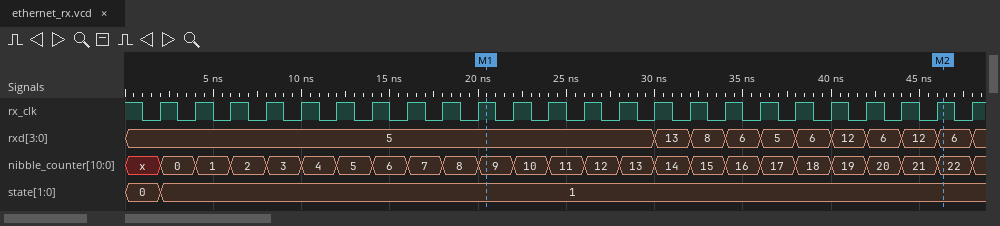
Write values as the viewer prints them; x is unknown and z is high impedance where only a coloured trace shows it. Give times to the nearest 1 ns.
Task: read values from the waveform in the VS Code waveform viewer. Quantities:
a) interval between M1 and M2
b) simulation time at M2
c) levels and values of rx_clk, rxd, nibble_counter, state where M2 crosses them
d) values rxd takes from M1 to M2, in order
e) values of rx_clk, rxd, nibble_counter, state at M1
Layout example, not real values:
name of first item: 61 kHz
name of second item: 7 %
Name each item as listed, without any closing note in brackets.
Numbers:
interval between M1 and M2: 26 ns
simulation time at M2: 46 ns
levels and values of rx_clk, rxd, nibble_counter, state where M2 crosses them: rx_clk=1, rxd=6, nibble_counter=22, state=1
values rxd takes from M1 to M2, in order: 5, 13, 8, 6, 5, 6, 12, 6, 12, 6
values of rx_clk, rxd, nibble_counter, state at M1: rx_clk=1, rxd=5, nibble_counter=9, state=1
